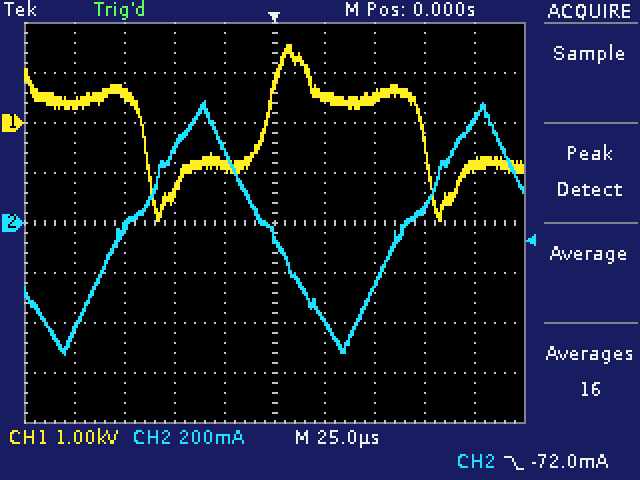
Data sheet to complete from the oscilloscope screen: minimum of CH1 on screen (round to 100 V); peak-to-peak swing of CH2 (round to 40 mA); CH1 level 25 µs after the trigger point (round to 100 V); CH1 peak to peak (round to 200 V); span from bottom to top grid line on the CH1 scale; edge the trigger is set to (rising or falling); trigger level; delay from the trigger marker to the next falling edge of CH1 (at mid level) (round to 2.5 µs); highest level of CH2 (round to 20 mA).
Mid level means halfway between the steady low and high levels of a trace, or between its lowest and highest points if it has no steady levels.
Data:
-2.0 kV
1.00 A
500 V
3.6 kV
8 kV
falling
-72.0 mA
75.0 µs
480 mA
